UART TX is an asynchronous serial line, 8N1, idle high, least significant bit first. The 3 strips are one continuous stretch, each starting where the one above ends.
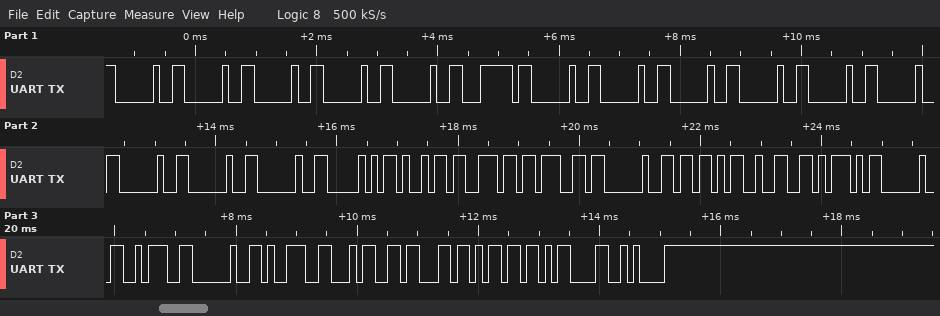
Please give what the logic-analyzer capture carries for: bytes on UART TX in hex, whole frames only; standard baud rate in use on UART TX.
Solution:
20 20 20 20 20 7C 20 20 20 20 20 20 20 20 20 50 69 6E 67 20 5B 32 5D 20 3A 20 39 34 63 6D 0D 0A
9600 baud
